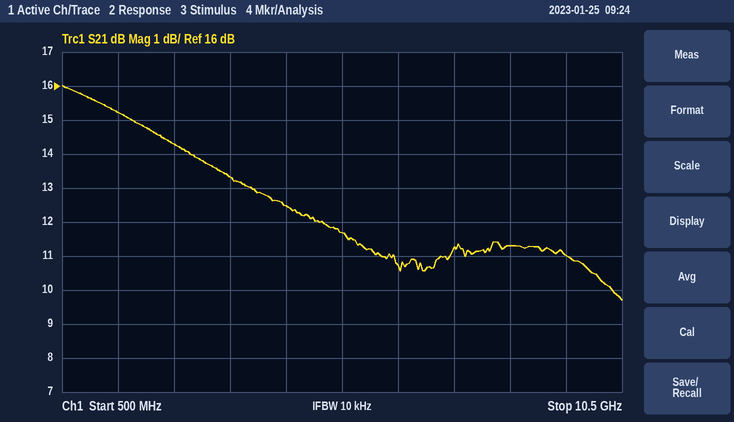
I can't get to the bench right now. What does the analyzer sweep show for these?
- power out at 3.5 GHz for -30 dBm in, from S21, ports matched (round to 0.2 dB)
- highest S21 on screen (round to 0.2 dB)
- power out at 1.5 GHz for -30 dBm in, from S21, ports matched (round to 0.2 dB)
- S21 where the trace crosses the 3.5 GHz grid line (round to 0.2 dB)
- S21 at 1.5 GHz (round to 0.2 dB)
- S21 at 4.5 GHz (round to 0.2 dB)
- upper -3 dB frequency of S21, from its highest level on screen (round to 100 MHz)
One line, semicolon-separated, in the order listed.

-16.6 dBm; 16.0 dB; -14.8 dBm; 13.4 dB; 15.2 dB; 12.4 dB; 3.9 GHz
